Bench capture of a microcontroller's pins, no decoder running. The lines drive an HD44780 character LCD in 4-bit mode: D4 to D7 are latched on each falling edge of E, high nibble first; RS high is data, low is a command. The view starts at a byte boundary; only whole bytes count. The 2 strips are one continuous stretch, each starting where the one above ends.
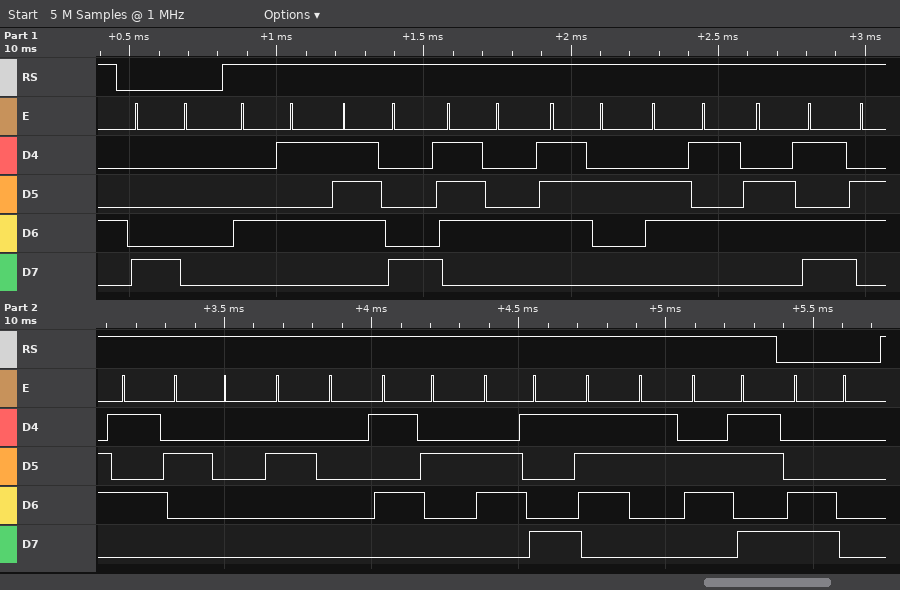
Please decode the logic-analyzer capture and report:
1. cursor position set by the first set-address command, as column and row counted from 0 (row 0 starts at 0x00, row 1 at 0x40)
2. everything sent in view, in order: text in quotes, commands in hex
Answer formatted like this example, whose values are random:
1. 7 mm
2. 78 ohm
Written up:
1. column 0, row 0
2. 0x80 "Extreme  Risk" 0xC0
